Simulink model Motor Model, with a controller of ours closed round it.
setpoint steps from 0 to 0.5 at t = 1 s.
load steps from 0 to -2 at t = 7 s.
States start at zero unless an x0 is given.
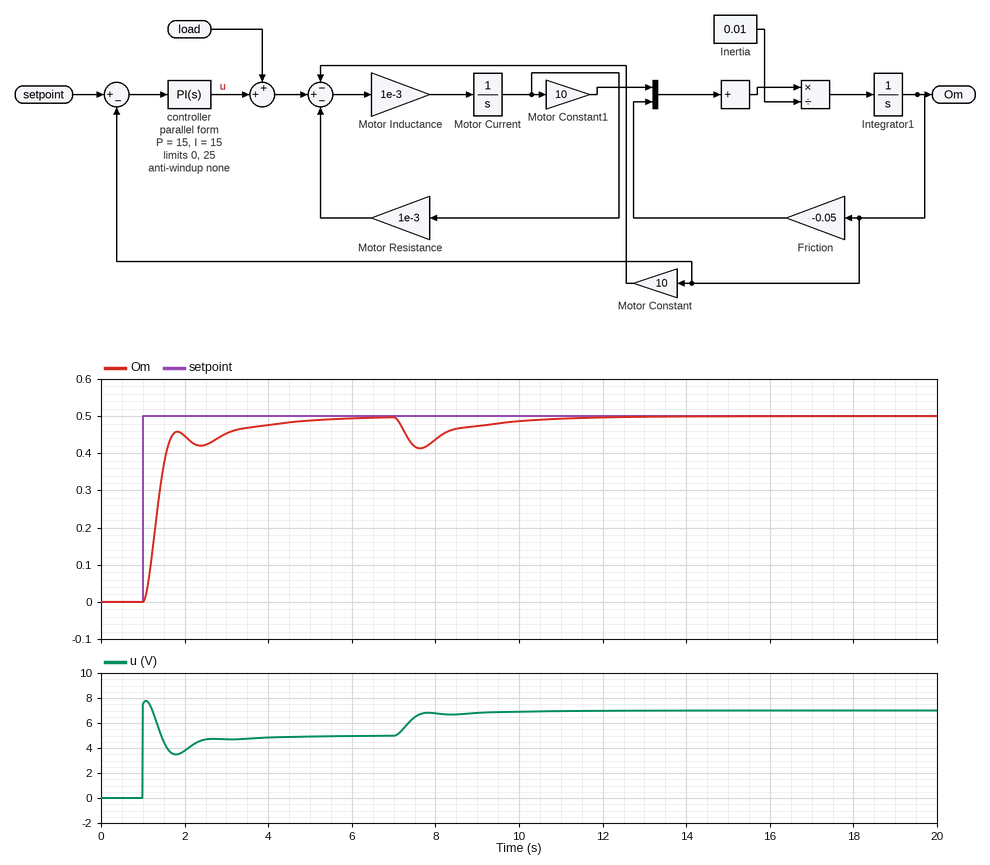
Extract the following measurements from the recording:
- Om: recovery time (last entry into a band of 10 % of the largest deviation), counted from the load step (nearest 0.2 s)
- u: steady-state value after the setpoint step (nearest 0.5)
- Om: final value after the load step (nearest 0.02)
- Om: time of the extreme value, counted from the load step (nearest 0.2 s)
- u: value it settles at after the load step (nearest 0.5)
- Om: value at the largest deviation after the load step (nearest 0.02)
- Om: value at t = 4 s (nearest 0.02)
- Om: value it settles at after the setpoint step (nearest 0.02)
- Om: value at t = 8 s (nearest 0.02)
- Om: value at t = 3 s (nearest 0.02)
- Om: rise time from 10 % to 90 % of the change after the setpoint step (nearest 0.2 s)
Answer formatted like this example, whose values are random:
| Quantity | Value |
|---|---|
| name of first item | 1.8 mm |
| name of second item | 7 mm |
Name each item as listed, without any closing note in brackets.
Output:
| Quantity | Value |
|---|---|
| Om: recovery time (last entry into a band of 10 % of the largest deviation), counted from the load step | 3.8 s |
| u: steady-state value after the setpoint step | 5.0 |
| Om: final value after the load step | 0.50 |
| Om: time of the extreme value, counted from the load step | 0.6 s |
| u: value it settles at after the load step | 7.0 |
| Om: value at the largest deviation after the load step | 0.42 |
| Om: value at t = 4 s | 0.48 |
| Om: value it settles at after the setpoint step | 0.50 |
| Om: value at t = 8 s | 0.44 |
| Om: value at t = 3 s | 0.46 |
| Om: rise time from 10 % to 90 % of the change after the setpoint step | 0.6 s |
